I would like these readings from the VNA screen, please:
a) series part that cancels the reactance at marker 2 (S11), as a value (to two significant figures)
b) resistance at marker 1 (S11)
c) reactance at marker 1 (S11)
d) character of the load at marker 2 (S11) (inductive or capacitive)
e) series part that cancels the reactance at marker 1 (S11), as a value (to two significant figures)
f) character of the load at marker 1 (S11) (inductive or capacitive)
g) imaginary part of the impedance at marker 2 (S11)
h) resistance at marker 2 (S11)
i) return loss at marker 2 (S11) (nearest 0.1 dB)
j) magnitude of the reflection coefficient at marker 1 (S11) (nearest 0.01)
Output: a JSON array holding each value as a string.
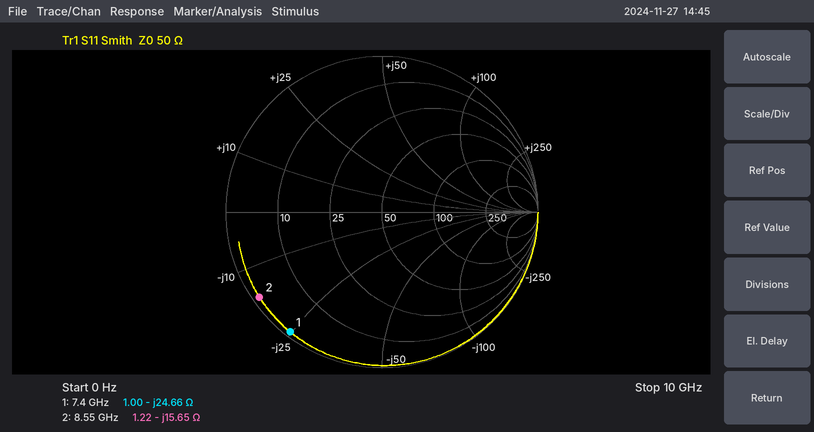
["290 pH", "1.00 Ω", "-24.66 Ω", "capacitive", "530 pH", "capacitive", "-15.65 Ω", "1.22 Ω", "0.4 dB", "0.97"]
